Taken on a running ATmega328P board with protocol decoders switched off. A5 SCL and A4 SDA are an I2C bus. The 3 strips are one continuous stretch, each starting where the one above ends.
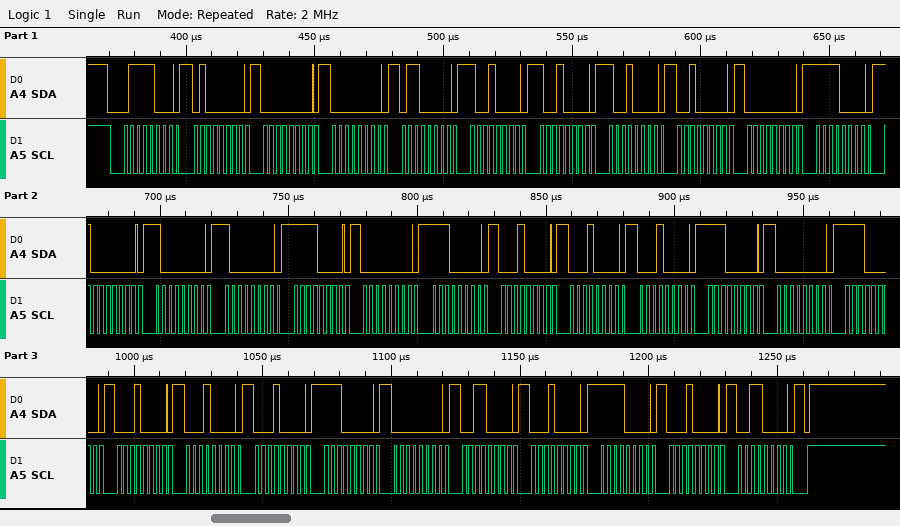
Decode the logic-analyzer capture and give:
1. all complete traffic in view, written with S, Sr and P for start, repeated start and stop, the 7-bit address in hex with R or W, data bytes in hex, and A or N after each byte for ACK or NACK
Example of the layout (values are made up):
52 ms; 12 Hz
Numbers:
S 3CW A 40 A 00 A 00 A 60 A 90 A 90 A 90 A 20 A 00 A F0 A 80 A 80 A 80 A F0 A 00 A E0 A 10 A 10 A 10 A E0 A 00 A E0 A 10 A 10 A 10 A E0 A 00 A 30 A 10 A F0 A 10 A 30 A P
